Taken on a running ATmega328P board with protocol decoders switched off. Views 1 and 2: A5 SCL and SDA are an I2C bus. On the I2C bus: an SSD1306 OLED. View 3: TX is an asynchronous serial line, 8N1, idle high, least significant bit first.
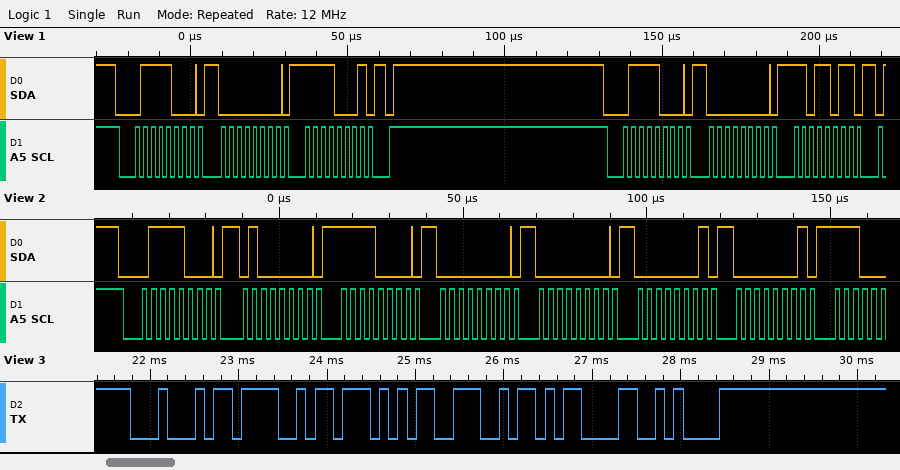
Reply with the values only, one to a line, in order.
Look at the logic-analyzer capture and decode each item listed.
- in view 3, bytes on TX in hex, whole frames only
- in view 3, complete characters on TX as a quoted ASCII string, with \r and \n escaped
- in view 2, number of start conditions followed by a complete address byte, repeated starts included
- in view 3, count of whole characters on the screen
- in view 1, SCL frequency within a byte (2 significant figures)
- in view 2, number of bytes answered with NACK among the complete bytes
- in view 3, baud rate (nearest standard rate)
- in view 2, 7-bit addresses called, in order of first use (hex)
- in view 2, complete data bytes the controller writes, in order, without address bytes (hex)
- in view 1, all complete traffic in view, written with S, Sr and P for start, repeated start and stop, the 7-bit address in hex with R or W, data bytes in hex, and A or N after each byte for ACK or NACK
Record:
44 4F 57 4E 0D 0A
"DOWN\r\n"
1
6
400 kHz
0
9600 baud
0x3C
40 F0 00 00 01 01
S 3CW A 00 A F1 A P S 3CW A 00 A DB A
